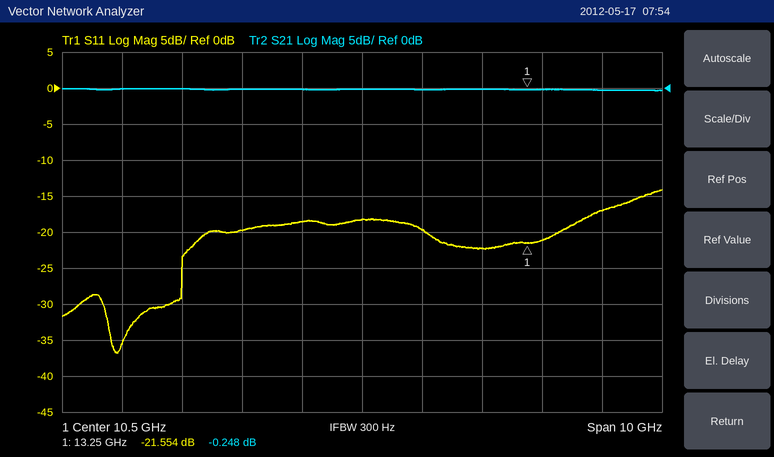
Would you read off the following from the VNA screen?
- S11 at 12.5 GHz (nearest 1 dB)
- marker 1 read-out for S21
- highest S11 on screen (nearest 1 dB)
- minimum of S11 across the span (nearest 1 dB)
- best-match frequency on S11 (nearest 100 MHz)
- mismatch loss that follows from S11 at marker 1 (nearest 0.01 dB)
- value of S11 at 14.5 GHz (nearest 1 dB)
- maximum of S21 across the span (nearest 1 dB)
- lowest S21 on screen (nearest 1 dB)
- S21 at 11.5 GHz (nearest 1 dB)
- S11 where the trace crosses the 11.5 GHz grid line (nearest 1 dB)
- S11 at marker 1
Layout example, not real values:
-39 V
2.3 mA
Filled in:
-22 dB
-0.248 dB
-14 dB
-37 dB
6.4 GHz
0.03 dB
-17 dB
0 dB
0 dB
0 dB
-20 dB
-21.554 dB
